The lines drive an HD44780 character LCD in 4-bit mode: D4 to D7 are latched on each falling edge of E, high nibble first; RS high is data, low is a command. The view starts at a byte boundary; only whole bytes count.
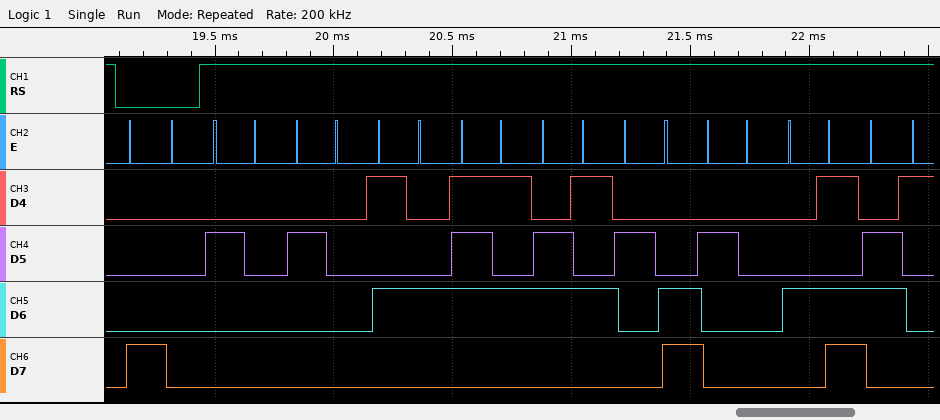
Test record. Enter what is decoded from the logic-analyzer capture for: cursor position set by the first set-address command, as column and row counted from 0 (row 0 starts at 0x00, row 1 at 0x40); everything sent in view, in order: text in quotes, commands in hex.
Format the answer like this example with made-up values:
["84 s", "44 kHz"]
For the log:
["column 0, row 0", "0x80 \"  Tue, Ma\""]
